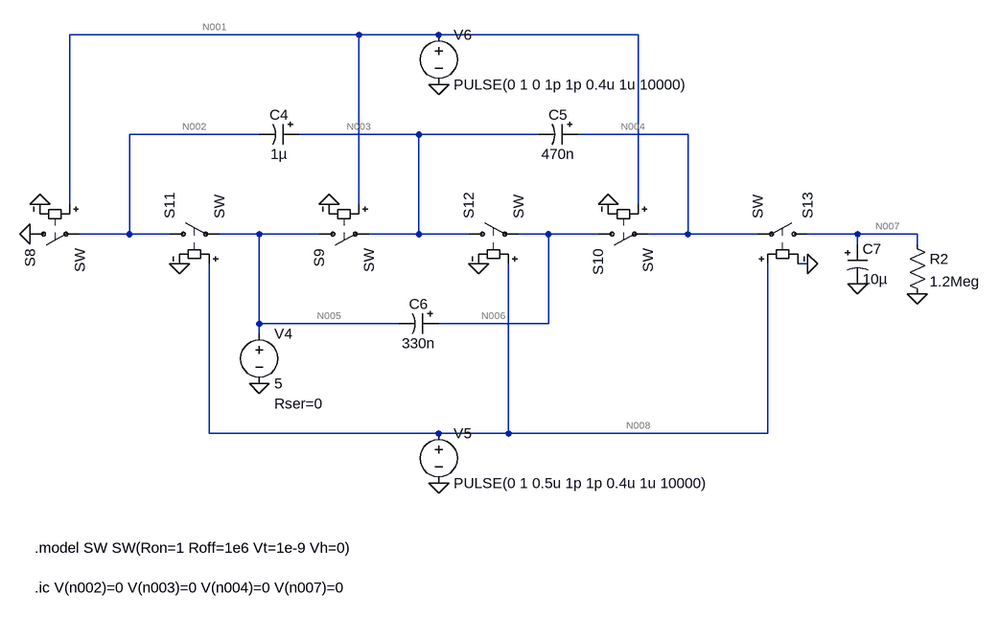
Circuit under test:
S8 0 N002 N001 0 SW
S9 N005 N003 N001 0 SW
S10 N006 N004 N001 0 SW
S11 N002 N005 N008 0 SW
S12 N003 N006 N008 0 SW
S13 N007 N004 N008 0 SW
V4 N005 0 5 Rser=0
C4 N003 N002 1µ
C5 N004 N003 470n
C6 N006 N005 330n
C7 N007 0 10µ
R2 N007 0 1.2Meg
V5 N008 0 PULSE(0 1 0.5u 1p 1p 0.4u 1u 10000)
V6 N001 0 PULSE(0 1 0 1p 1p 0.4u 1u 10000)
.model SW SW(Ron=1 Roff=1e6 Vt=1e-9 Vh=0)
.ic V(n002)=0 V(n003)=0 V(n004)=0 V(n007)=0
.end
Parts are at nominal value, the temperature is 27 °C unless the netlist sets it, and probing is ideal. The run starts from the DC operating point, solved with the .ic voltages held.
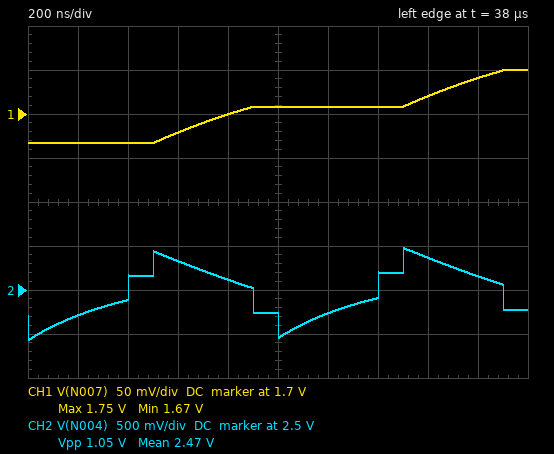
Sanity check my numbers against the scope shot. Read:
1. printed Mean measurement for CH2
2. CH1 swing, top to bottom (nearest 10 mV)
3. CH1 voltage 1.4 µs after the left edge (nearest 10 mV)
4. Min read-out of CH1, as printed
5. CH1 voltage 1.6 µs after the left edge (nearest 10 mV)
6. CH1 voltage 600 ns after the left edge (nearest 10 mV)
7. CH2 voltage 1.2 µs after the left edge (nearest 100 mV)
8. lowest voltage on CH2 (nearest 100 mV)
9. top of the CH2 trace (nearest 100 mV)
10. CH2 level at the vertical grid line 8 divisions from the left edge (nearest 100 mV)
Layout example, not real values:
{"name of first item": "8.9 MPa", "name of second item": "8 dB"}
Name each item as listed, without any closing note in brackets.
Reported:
{"printed Mean measurement for CH2": "2.47 V", "CH1 swing, top to bottom": "80 mV", "CH1 voltage 1.4 µs after the left edge": "1.71 V", "Min read-out of CH1, as printed": "1.67 V", "CH1 voltage 1.6 µs after the left edge": "1.72 V", "CH1 voltage 600 ns after the left edge": "1.68 V", "CH2 voltage 1.2 µs after the left edge": "2.2 V", "lowest voltage on CH2": "1.9 V", "top of the CH2 trace": "3.0 V", "CH2 level at the vertical grid line 8 divisions from the left edge": "2.9 V"}
